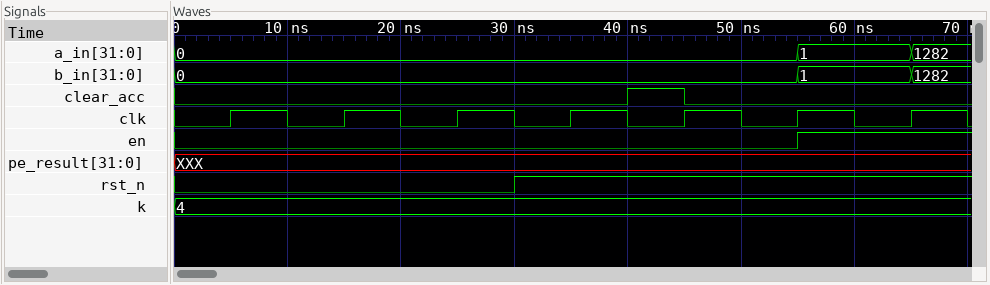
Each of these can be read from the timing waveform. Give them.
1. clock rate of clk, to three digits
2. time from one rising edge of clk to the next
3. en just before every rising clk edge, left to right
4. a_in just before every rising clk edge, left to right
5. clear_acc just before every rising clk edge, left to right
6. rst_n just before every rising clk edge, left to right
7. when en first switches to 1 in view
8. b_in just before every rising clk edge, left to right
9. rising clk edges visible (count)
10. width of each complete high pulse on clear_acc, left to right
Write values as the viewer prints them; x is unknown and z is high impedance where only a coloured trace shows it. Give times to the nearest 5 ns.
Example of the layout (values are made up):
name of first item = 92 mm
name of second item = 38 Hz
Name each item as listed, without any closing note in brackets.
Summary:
clock rate of clk, to three digits = 100 MHz
time from one rising edge of clk to the next = 10 ns
en just before every rising clk edge, left to right = 0 0 0 0 0 0 1
a_in just before every rising clk edge, left to right = 0, 0, 0, 0, 0, 0, 1
clear_acc just before every rising clk edge, left to right = 0 0 0 0 1 0 0
rst_n just before every rising clk edge, left to right = 0 0 0 1 1 1 1
when en first switches to 1 in view = 55 ns
b_in just before every rising clk edge, left to right = 0, 0, 0, 0, 0, 0, 1
rising clk edges visible = 7
width of each complete high pulse on clear_acc, left to right = 5 ns
